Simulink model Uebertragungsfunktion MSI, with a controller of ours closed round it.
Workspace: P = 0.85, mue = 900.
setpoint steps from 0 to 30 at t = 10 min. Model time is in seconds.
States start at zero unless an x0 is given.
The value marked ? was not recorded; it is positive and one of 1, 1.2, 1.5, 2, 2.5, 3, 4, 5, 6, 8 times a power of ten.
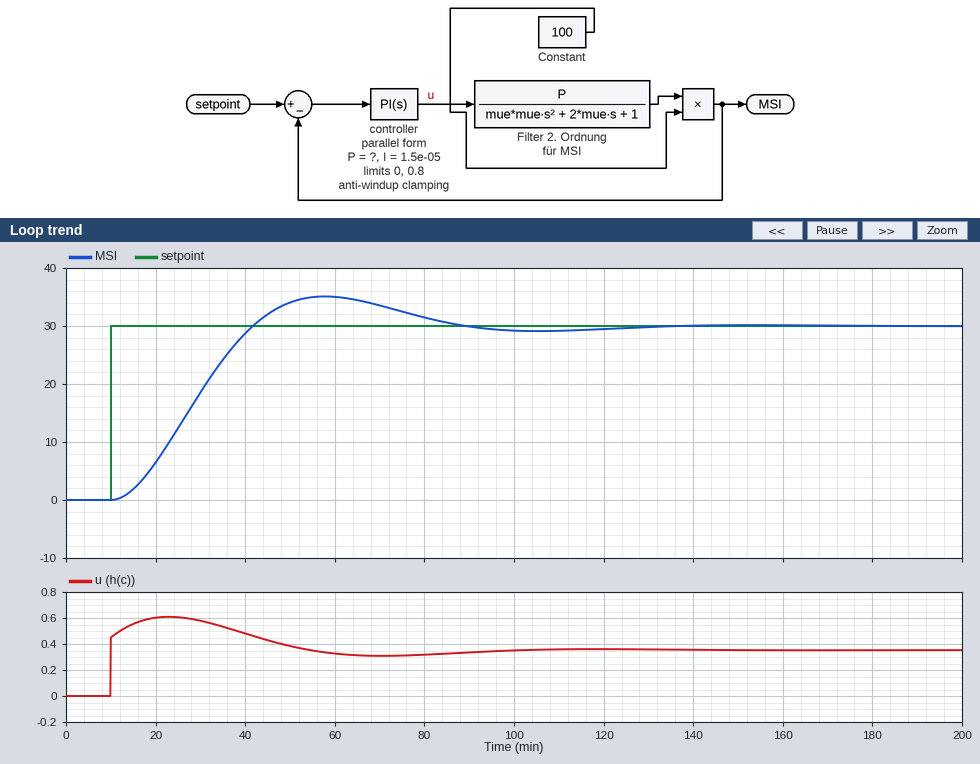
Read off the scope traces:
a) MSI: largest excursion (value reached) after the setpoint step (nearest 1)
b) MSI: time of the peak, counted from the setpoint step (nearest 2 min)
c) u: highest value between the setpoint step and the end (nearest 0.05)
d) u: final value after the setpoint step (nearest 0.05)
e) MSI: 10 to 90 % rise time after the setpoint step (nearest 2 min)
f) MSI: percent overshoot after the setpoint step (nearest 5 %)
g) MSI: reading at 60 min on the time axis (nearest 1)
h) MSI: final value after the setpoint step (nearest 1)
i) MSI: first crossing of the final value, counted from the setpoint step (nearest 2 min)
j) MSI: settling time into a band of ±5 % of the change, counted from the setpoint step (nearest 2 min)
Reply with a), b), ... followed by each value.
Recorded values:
a) 35
b) 48 min
c) 0.60
d) 0.35
e) 22 min
f) 15 %
g) 35
h) 30
i) 32 min
j) 70 min
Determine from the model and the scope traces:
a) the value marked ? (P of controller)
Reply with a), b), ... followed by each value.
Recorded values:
a) 0.015
